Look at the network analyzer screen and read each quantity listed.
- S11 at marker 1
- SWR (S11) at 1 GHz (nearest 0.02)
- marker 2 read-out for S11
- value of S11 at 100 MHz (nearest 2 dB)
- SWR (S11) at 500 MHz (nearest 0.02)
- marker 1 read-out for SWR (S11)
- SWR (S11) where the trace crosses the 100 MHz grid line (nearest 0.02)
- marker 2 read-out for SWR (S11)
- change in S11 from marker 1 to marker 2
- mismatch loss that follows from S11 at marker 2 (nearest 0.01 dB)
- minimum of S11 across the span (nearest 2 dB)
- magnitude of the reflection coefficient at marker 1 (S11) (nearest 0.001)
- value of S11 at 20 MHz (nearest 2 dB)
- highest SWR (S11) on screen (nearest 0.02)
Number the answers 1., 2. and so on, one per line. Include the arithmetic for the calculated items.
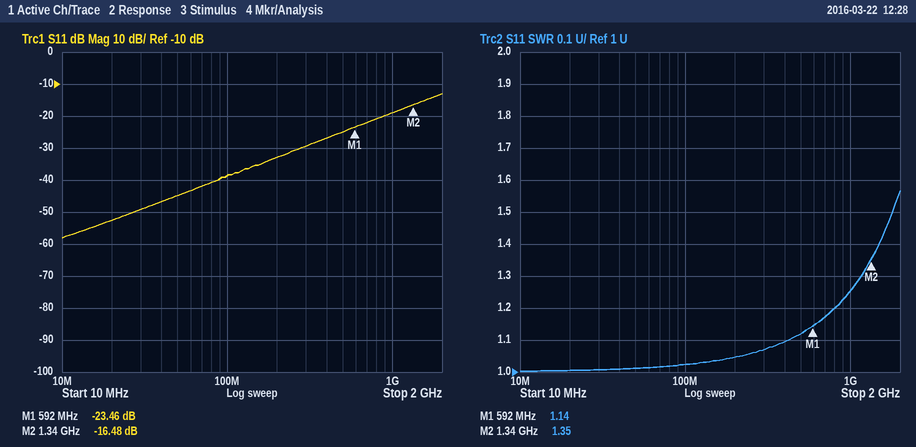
1. -23.46 dB
2. 1.26
3. -16.48 dB
4. -38 dB
5. 1.12
6. 1.14
7. 1.02
8. 1.35
9. -16.48 − (-23.46) = 6.98 dB
10. −10 log10(1 − 10^(-16.48/10)) ≈ 0.10 dB
11. -58 dB
12. 10^(-23.46/20) ≈ 0.067
13. -52 dB
14. 1.56
